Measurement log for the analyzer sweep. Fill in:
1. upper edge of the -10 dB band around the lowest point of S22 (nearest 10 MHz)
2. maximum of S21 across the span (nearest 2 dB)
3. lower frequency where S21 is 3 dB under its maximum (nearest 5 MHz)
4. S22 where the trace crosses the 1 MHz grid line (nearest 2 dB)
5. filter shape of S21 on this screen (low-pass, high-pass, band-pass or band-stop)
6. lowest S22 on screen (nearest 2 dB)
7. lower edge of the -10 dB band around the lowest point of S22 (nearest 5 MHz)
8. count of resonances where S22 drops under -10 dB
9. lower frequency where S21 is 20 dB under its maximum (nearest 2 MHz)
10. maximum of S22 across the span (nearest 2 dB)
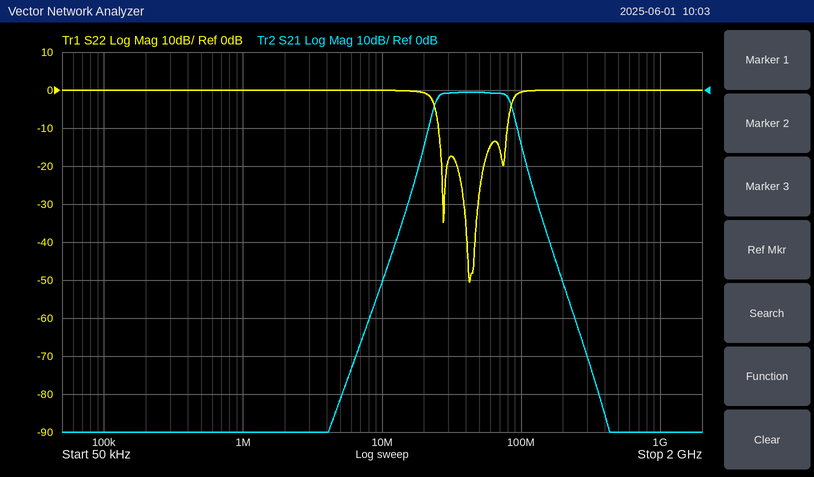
80 MHz
0 dB
25 MHz
0 dB
band-pass
-50 dB
25 MHz
3
18 MHz
0 dB
